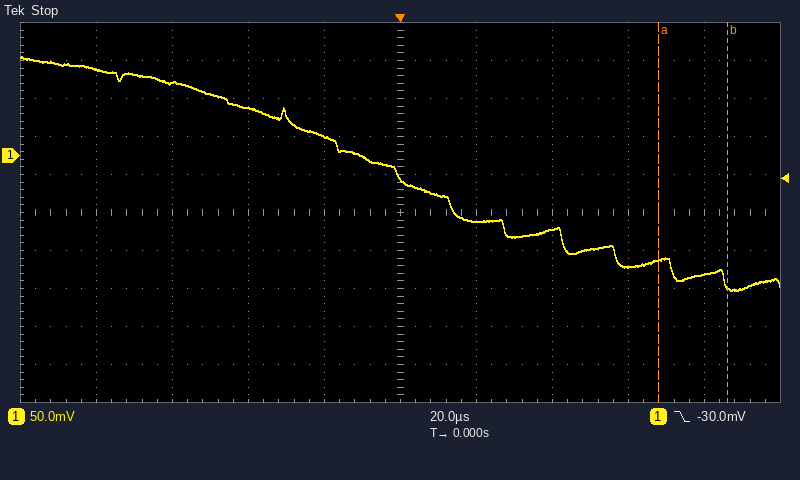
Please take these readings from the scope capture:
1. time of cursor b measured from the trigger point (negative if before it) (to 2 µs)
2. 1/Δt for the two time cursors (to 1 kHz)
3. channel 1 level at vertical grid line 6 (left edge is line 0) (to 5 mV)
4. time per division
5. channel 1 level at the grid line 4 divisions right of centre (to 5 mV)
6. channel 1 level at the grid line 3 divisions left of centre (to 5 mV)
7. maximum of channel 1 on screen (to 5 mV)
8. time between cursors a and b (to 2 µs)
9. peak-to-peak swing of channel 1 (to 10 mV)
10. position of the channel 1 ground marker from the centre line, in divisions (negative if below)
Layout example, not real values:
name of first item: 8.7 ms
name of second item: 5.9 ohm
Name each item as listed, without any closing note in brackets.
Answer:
time of cursor b measured from the trigger point (negative if before it): +86 µs
1/Δt for the two time cursors: 56 kHz
channel 1 level at vertical grid line 6 (left edge is line 0): -85 mV
time per division: 20 µs
channel 1 level at the grid line 4 divisions right of centre: -155 mV
channel 1 level at the grid line 3 divisions left of centre: 95 mV
maximum of channel 1 on screen: 130 mV
time between cursors a and b: 18 µs
peak-to-peak swing of channel 1: 310 mV
position of the channel 1 ground marker from the centre line, in divisions: +1.5 div
